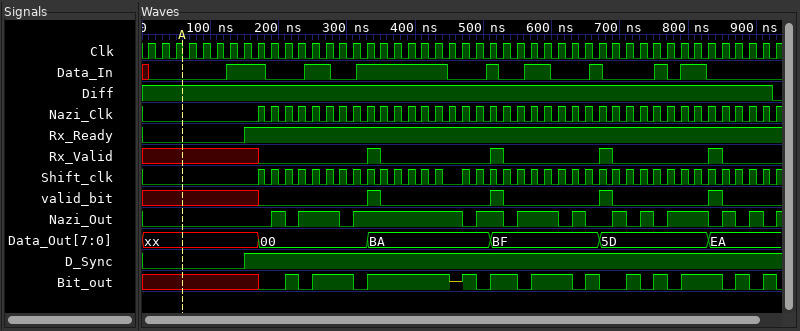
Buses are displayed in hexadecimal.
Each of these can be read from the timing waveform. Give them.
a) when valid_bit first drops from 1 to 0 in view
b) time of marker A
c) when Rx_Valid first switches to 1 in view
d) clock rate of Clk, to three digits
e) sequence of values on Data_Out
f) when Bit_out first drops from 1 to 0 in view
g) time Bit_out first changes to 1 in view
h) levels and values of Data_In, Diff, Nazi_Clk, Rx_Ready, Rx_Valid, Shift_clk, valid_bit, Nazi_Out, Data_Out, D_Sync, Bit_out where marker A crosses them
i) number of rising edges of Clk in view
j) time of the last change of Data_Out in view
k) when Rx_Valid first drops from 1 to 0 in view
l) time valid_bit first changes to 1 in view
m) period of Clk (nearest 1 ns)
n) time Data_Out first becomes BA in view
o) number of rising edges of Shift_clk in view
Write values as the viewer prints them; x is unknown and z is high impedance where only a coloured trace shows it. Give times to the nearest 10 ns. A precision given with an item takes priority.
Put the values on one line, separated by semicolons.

350 ns; 60 ns; 330 ns; 50.0 MHz; xx, 00, BA, BF, 5D, EA; 230 ns; 210 ns; Data_In=0, Diff=1, Nazi_Clk=0, Rx_Ready=0, Rx_Valid=x, Shift_clk=0, valid_bit=x, Nazi_Out=0, Data_Out=xx, D_Sync=0, Bit_out=x; 47; 830 ns; 350 ns; 330 ns; 20 ns; 330 ns; 38
